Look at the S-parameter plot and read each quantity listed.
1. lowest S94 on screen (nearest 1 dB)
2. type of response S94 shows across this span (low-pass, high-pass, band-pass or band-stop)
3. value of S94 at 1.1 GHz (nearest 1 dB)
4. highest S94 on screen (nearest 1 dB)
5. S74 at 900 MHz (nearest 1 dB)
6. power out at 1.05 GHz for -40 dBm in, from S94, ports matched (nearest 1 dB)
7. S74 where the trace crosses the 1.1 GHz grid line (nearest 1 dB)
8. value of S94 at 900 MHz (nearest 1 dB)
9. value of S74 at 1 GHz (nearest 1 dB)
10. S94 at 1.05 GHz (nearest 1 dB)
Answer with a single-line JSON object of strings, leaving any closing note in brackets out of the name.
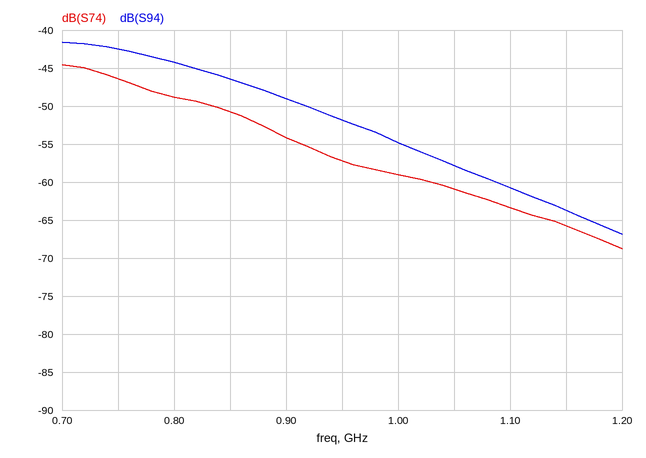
{"lowest S94 on screen": "-67 dB", "type of response S94 shows across this span": "low-pass", "value of S94 at 1.1 GHz": "-61 dB", "highest S94 on screen": "-42 dB", "S74 at 900 MHz": "-54 dB", "power out at 1.05 GHz for -40 dBm in, from S94, ports matched": "-98 dBm", "S74 where the trace crosses the 1.1 GHz grid line": "-63 dB", "value of S94 at 900 MHz": "-49 dB", "value of S74 at 1 GHz": "-59 dB", "S94 at 1.05 GHz": "-58 dB"}
